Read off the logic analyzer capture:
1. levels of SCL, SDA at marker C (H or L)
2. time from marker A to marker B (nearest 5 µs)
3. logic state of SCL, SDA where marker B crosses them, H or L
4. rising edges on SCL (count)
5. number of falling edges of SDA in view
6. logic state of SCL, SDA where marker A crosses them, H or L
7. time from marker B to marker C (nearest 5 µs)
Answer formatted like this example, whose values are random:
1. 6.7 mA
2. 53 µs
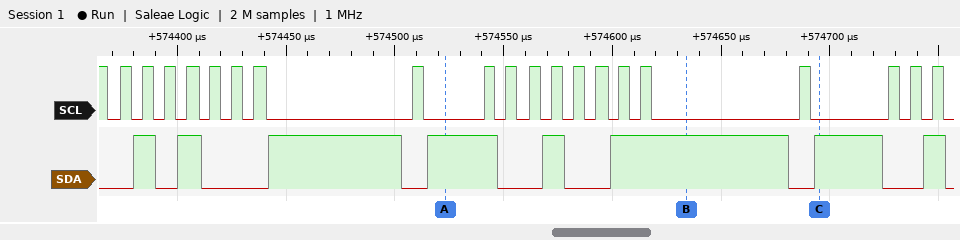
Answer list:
1. SCL=L, SDA=H
2. 110 µs
3. SCL=L, SDA=H
4. 20
5. 8
6. SCL=L, SDA=H
7. 60 µs
